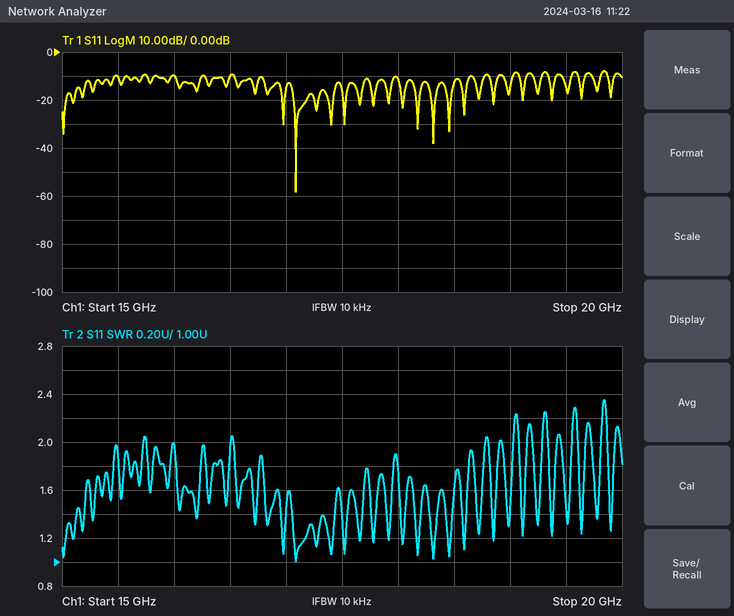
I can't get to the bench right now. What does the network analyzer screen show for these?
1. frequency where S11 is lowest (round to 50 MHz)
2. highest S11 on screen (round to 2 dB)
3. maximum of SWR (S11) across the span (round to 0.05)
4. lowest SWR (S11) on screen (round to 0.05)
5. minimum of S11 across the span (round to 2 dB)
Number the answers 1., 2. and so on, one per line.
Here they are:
1. 17.10 GHz
2. -8 dB
3. 2.35
4. 1.00
5. -58 dB
